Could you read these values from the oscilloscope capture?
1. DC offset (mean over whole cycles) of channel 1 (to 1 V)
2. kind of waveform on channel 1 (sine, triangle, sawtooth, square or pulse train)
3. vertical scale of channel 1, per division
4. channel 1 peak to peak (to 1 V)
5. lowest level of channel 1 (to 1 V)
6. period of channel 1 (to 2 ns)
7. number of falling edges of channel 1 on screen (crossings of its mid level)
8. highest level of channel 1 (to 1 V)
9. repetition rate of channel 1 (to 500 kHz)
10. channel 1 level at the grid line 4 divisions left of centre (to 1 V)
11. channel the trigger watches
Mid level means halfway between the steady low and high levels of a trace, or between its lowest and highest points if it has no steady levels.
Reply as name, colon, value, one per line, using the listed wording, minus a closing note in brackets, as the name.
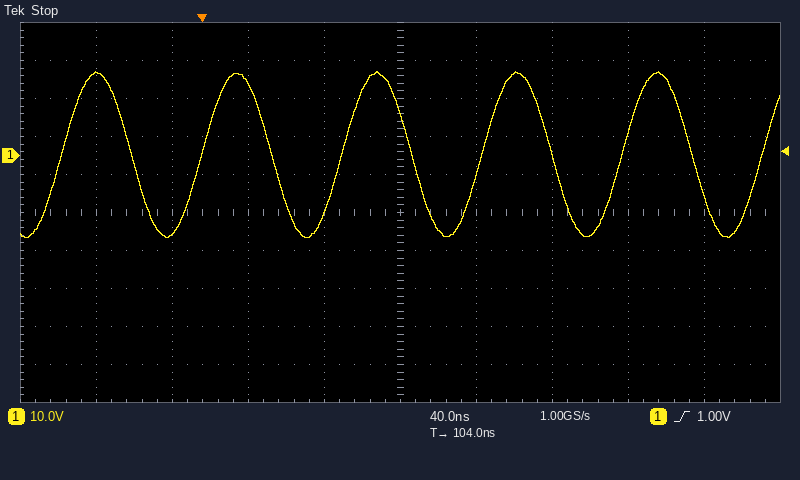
DC offset (mean over whole cycles) of channel 1: 0 V
kind of waveform on channel 1: sine
vertical scale of channel 1, per division: 10 V
channel 1 peak to peak: 44 V
lowest level of channel 1: -22 V
period of channel 1: 74 ns
number of falling edges of channel 1 on screen: 5
highest level of channel 1: 22 V
repetition rate of channel 1: 13.5 MHz
channel 1 level at the grid line 4 divisions left of centre: 22 V
channel the trigger watches: channel 1
